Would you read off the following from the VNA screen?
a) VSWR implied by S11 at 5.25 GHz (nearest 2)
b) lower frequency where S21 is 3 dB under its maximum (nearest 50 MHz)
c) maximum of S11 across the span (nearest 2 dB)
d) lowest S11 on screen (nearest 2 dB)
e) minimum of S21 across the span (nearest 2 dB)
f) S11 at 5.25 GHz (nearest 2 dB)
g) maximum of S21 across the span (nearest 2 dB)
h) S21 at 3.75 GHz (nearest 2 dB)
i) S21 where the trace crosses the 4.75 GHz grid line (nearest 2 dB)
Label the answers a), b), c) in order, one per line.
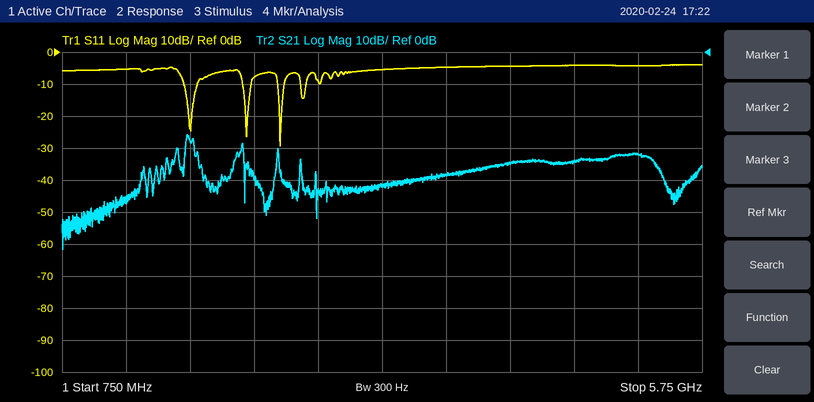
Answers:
a) 4
b) 1.70 GHz
c) -4 dB
d) -30 dB
e) -62 dB
f) -4 dB
g) -26 dB
h) -38 dB
i) -34 dB
